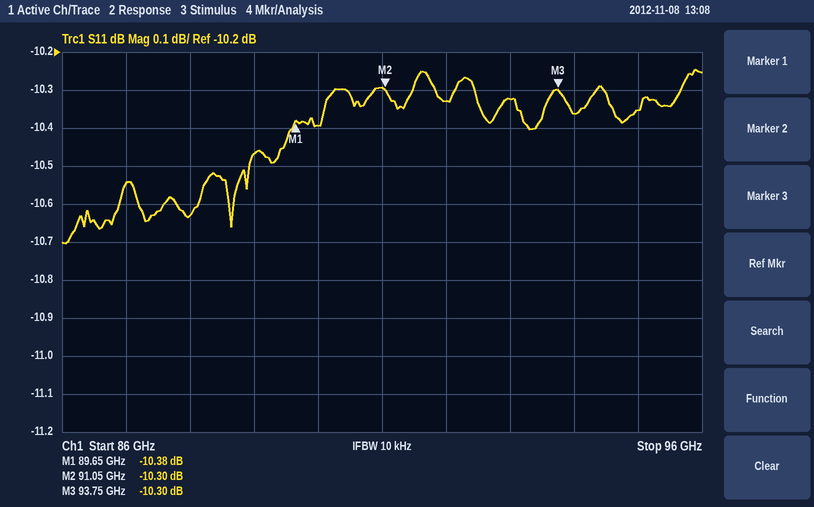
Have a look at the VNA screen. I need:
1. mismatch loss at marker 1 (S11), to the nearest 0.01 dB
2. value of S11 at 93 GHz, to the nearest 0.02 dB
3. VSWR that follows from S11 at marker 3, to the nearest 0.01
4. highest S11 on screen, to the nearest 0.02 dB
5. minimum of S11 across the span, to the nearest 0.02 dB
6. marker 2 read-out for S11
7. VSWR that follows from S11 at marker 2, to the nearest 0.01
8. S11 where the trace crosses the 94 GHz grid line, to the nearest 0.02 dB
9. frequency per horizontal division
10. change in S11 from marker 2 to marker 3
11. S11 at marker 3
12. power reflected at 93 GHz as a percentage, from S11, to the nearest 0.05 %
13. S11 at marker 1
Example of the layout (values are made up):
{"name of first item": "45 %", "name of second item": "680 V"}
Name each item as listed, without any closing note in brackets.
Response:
{"mismatch loss at marker 1 (S11), to the nearest 0.01 dB": "0.42 dB", "value of S11 at 93 GHz, to the nearest 0.02 dB": "-10.32 dB", "VSWR that follows from S11 at marker 3, to the nearest 0.01": "1.88", "highest S11 on screen, to the nearest 0.02 dB": "-10.24 dB", "minimum of S11 across the span, to the nearest 0.02 dB": "-10.70 dB", "marker 2 read-out for S11": "-10.30 dB", "VSWR that follows from S11 at marker 2, to the nearest 0.01": "1.88", "S11 where the trace crosses the 94 GHz grid line, to the nearest 0.02 dB": "-10.36 dB", "frequency per horizontal division": "1 GHz", "change in S11 from marker 2 to marker 3": "0.00 dB", "S11 at marker 3": "-10.30 dB", "power reflected at 93 GHz as a percentage, from S11, to the nearest 0.05 %": "9.30 %", "S11 at marker 1": "-10.38 dB"}
